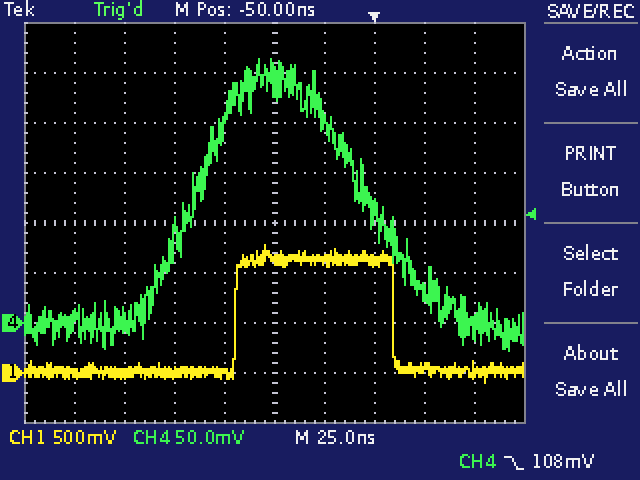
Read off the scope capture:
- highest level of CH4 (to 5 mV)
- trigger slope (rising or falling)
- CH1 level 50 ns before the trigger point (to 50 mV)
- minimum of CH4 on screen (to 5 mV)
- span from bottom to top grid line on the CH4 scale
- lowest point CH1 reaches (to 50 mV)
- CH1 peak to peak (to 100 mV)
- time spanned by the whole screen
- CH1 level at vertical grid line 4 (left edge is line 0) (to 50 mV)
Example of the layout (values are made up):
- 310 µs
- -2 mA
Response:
- 265 mV
- falling
- 1.15 V
- -30 mV
- 400 mV
- -100 mV
- 1.40 V
- 250 ns
- 0 mV
